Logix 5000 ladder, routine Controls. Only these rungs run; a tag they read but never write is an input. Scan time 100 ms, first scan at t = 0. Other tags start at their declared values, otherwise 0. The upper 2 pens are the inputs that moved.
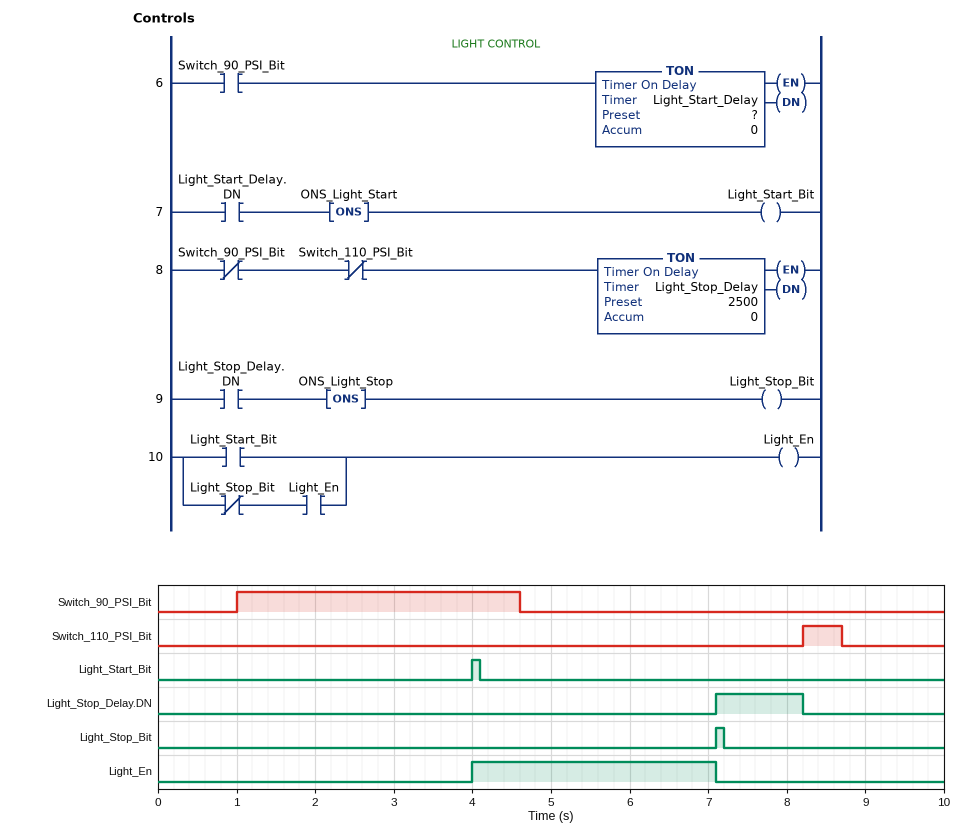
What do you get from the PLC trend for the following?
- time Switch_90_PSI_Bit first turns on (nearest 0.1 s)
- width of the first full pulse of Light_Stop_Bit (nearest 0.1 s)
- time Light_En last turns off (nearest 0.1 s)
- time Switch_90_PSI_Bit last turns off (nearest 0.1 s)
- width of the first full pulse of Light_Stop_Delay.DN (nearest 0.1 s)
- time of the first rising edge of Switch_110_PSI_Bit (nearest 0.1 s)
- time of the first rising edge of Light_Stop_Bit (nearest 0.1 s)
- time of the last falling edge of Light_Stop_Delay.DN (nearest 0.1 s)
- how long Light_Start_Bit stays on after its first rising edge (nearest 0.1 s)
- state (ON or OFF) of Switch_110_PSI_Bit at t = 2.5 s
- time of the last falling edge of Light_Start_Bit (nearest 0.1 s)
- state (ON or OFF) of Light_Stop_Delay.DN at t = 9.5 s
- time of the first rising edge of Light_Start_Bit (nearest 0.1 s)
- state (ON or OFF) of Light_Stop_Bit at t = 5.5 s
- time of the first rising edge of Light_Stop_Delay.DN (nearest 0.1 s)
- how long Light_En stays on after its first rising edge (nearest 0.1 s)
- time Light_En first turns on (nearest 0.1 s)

1.0 s
0.1 s
7.1 s
4.6 s
1.1 s
8.2 s
7.1 s
8.2 s
0.1 s
OFF
4.1 s
OFF
4.0 s
OFF
7.1 s
3.1 s
4.0 s
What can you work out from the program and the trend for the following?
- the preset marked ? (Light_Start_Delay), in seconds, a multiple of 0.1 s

3.0 s
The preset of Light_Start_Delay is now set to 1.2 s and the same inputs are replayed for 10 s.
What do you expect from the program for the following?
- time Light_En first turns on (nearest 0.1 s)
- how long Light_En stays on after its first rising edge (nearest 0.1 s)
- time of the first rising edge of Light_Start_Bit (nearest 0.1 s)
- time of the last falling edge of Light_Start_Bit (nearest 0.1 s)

2.2 s
4.9 s
2.2 s
2.3 s
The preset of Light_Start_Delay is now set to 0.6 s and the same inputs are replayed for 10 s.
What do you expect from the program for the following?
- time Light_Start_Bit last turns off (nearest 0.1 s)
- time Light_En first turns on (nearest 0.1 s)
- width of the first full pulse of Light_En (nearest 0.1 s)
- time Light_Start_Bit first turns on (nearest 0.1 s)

1.7 s
1.6 s
5.5 s
1.6 s
